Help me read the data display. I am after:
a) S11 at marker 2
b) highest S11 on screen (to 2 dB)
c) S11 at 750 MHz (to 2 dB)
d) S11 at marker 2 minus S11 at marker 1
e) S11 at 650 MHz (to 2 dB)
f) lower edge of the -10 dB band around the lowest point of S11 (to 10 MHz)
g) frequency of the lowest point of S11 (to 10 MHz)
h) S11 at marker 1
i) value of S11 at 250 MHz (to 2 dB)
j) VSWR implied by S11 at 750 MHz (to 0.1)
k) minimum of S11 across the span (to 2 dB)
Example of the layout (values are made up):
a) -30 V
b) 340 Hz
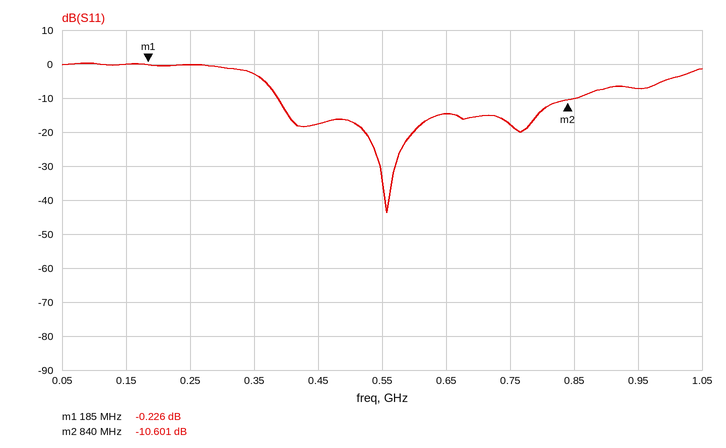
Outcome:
a) -10.601 dB
b) 0 dB
c) -18 dB
d) -10.375 dB
e) -14 dB
f) 390 MHz
g) 560 MHz
h) -0.226 dB
i) 0 dB
j) 1.3
k) -44 dB
